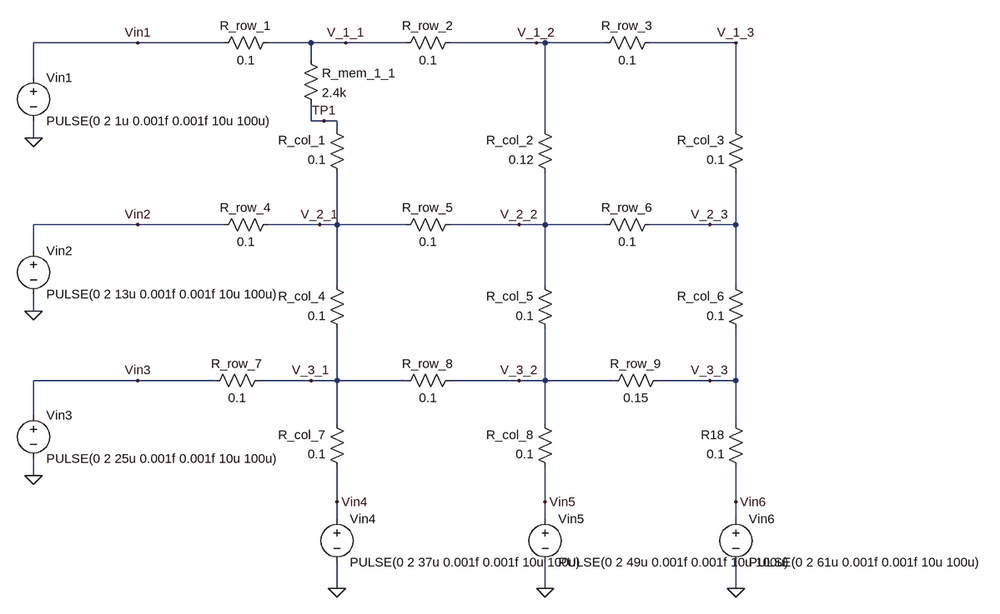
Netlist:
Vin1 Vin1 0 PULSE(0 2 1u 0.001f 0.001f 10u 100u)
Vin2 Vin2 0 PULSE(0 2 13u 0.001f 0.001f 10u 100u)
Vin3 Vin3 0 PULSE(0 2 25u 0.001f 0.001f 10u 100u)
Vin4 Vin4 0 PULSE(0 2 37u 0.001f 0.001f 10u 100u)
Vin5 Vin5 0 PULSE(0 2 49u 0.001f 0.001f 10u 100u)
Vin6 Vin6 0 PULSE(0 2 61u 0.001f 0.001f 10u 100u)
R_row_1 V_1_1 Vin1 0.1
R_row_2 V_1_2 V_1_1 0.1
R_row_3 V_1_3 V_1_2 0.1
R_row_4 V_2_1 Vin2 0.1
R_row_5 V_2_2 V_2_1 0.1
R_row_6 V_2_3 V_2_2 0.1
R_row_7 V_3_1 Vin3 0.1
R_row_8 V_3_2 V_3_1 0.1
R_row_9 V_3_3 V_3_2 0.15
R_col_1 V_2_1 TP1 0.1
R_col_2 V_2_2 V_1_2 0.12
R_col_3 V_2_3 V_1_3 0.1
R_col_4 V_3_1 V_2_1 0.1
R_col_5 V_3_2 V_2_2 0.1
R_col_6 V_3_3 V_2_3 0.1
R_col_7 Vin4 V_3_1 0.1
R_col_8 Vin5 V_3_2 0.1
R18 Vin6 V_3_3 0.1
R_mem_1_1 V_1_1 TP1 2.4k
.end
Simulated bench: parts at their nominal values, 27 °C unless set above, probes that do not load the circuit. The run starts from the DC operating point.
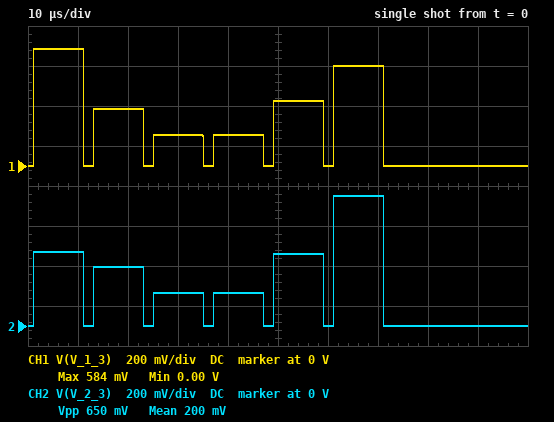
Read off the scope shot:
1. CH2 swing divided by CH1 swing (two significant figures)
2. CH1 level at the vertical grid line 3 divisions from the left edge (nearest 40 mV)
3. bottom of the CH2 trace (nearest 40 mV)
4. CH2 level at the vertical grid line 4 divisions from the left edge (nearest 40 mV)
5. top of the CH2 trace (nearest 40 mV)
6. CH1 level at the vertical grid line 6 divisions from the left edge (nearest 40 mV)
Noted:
1.1
160 mV
0 V
160 mV
640 mV
0 V
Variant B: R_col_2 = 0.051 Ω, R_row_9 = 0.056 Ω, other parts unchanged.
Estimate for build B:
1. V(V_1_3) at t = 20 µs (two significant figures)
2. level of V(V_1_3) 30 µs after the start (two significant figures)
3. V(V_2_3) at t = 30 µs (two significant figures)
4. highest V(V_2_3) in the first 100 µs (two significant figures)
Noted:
310 mV
170 mV
180 mV
580 mV
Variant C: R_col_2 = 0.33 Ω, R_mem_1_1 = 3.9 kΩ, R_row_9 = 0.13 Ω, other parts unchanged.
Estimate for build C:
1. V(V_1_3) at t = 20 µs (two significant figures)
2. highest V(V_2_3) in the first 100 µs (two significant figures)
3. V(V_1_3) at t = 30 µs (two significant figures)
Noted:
260 mV
640 mV
140 mV
